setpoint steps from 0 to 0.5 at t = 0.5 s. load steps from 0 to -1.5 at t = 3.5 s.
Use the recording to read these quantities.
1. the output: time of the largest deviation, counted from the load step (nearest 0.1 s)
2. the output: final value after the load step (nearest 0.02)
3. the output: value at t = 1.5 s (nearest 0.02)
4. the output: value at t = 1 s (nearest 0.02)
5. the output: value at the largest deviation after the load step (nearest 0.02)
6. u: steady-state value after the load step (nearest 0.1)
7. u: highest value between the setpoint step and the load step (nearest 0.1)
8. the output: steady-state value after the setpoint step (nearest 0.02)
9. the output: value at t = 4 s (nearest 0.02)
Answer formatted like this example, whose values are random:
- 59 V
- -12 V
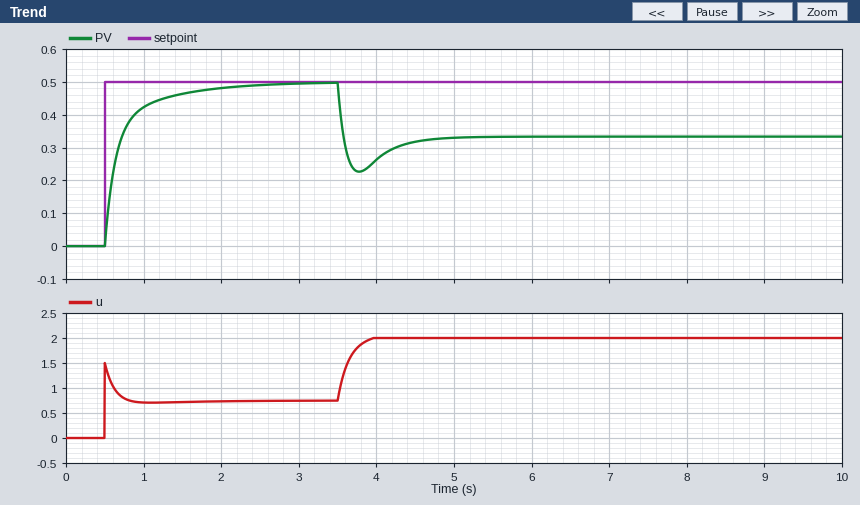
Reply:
- 0.3 s
- 0.34
- 0.46
- 0.42
- 0.22
- 2.0
- 1.5
- 0.50
- 0.26
